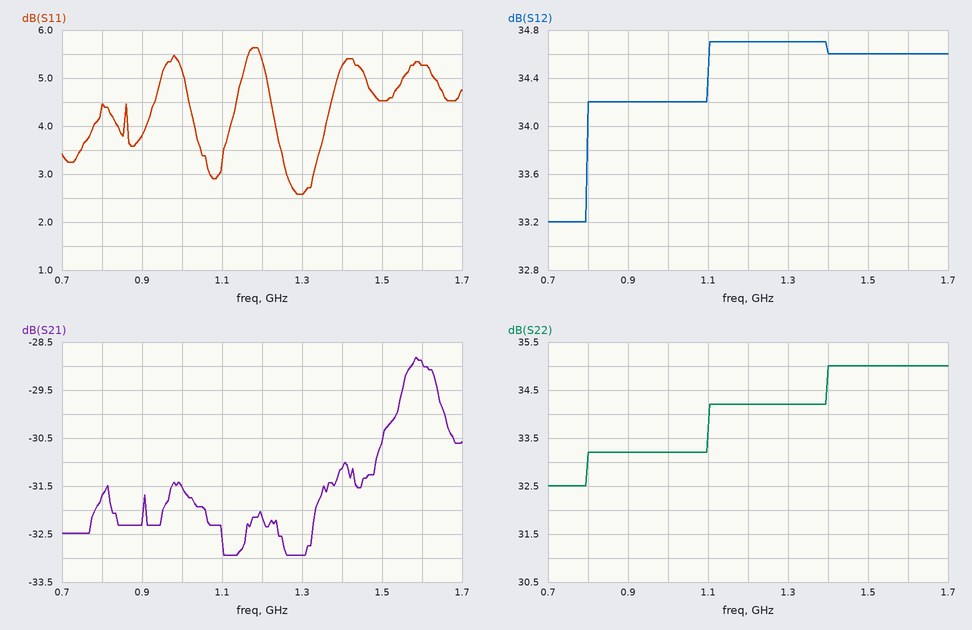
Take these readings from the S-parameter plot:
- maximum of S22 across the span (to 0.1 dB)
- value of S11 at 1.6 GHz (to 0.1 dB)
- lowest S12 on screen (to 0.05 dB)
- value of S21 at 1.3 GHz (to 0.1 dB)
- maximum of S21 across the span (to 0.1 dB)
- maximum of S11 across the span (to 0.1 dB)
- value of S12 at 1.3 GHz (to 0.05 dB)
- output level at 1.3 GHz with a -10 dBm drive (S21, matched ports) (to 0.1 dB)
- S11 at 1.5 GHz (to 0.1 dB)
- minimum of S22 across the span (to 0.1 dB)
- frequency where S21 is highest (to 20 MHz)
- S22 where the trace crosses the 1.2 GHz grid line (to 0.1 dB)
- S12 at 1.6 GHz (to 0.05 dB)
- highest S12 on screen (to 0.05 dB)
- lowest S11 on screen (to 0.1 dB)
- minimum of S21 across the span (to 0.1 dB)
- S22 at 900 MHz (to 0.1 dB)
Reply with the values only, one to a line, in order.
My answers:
35.0 dB
5.3 dB
33.20 dB
-32.9 dB
-28.8 dB
5.6 dB
34.70 dB
-42.9 dBm
4.5 dB
32.5 dB
1.58 GHz
34.2 dB
34.60 dB
34.70 dB
2.6 dB
-32.9 dB
33.2 dB
